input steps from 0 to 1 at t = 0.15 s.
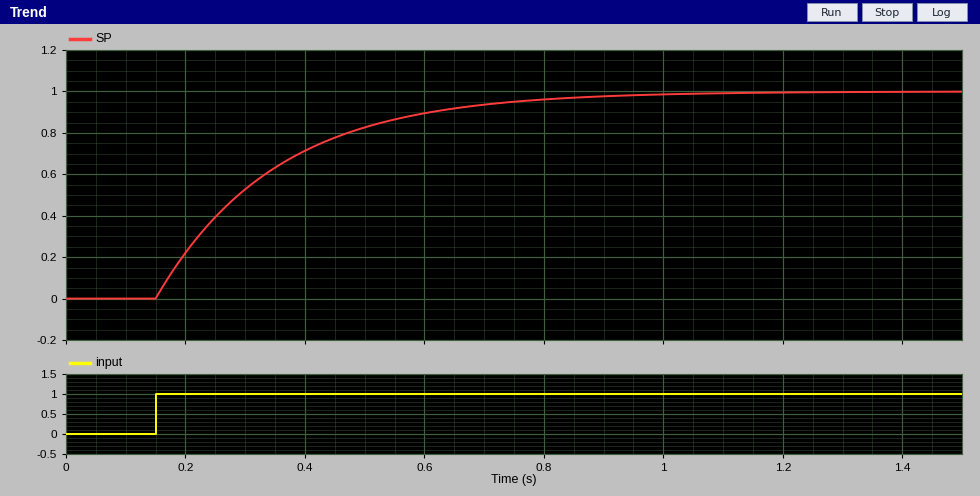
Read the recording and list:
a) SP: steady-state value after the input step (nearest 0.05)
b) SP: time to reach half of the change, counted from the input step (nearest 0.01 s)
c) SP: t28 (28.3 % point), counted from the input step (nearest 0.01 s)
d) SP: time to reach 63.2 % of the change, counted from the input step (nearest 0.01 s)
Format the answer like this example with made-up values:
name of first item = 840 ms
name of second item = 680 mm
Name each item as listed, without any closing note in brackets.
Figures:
SP: steady-state value after the input step = 1.00
SP: time to reach half of the change, counted from the input step = 0.14 s
SP: t28 (28.3 % point), counted from the input step = 0.07 s
SP: time to reach 63.2 % of the change, counted from the input step = 0.20 s
